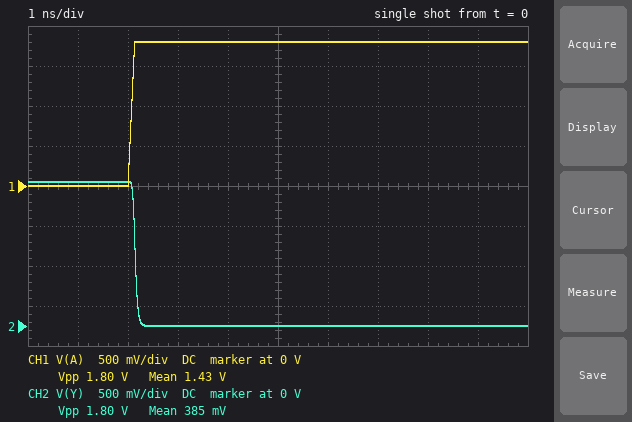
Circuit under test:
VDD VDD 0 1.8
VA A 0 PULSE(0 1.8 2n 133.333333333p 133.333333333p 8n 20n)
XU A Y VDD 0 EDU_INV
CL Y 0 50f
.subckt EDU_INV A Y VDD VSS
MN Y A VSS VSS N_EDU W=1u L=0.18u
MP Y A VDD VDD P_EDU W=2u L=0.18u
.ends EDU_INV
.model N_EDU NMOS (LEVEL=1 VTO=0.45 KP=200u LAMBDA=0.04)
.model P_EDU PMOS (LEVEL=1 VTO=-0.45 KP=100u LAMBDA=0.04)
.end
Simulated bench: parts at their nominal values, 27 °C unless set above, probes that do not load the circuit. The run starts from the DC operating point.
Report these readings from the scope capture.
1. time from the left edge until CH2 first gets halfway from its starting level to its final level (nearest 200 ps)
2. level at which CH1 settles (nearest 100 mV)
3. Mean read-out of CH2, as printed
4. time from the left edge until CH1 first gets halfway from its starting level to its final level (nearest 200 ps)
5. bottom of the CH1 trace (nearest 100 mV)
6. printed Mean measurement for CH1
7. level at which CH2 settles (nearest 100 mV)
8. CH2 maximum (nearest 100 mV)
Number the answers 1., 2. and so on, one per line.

1. 2.2 ns
2. 1.8 V
3. 385 mV
4. 2.0 ns
5. 0 V
6. 1.43 V
7. 0 V
8. 1.8 V
